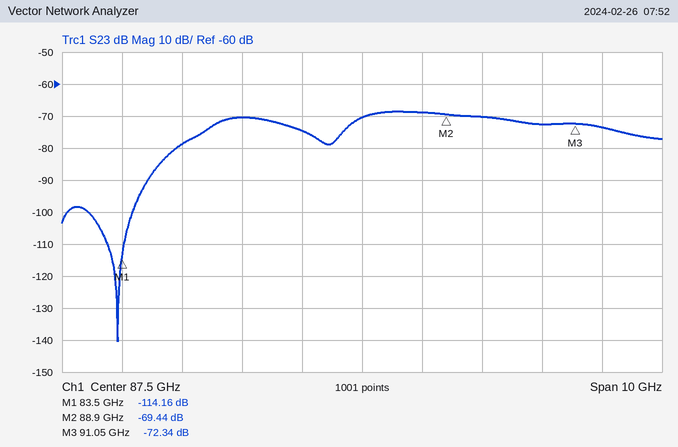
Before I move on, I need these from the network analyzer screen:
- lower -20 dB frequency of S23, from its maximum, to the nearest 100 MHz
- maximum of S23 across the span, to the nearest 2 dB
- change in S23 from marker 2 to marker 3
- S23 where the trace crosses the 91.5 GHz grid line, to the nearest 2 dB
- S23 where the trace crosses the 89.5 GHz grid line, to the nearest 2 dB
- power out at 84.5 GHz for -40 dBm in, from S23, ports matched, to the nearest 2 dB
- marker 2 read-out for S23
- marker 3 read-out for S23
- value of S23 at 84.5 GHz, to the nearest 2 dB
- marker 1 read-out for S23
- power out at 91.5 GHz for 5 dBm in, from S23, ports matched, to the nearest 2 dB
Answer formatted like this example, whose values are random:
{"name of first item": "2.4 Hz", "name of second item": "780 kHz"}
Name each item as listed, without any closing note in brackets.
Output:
{"lower -20 dB frequency of S23, from its maximum, to the nearest 100 MHz": "84.0 GHz", "maximum of S23 across the span, to the nearest 2 dB": "-68 dB", "change in S23 from marker 2 to marker 3": "-2.90 dB", "S23 where the trace crosses the 91.5 GHz grid line, to the nearest 2 dB": "-74 dB", "S23 where the trace crosses the 89.5 GHz grid line, to the nearest 2 dB": "-70 dB", "power out at 84.5 GHz for -40 dBm in, from S23, ports matched, to the nearest 2 dB": "-118 dBm", "marker 2 read-out for S23": "-69.44 dB", "marker 3 read-out for S23": "-72.34 dB", "value of S23 at 84.5 GHz, to the nearest 2 dB": "-78 dB", "marker 1 read-out for S23": "-114.16 dB", "power out at 91.5 GHz for 5 dBm in, from S23, ports matched, to the nearest 2 dB": "-68 dBm"}
